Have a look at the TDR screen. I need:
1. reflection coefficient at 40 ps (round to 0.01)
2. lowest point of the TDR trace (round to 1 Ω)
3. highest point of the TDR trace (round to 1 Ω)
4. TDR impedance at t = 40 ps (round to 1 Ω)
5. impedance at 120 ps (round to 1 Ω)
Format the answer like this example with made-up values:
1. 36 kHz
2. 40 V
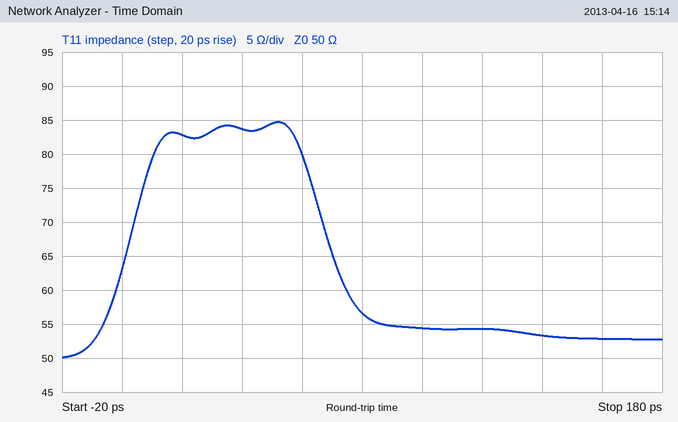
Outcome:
1. +0.25
2. 50 Ω
3. 85 Ω
4. 84 Ω
5. 54 Ω
